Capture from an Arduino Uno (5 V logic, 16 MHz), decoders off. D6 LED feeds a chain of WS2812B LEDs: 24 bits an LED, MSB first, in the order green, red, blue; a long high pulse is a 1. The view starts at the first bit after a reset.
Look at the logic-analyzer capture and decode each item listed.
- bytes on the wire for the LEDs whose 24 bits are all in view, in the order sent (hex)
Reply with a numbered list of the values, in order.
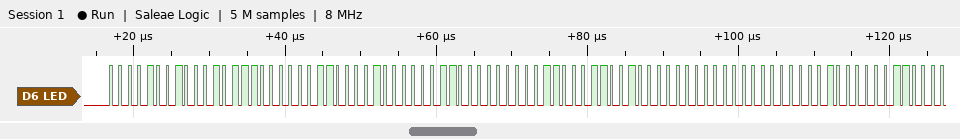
1. 09 17 03 08 18 03 19 00 00
